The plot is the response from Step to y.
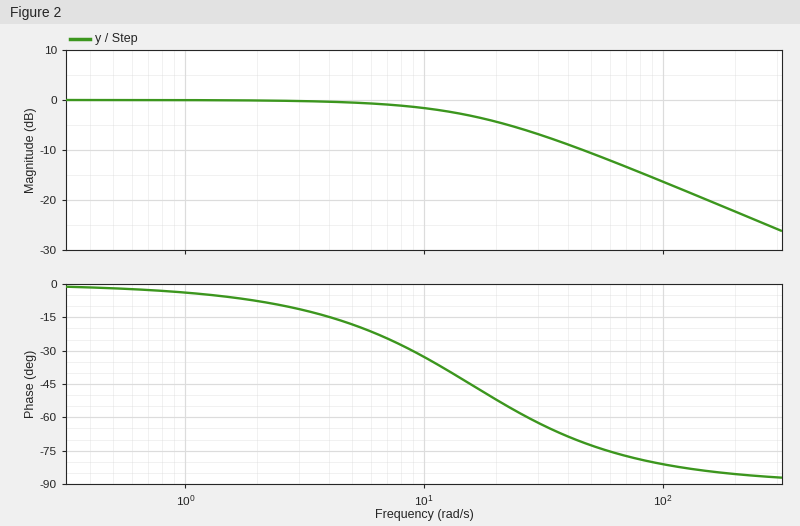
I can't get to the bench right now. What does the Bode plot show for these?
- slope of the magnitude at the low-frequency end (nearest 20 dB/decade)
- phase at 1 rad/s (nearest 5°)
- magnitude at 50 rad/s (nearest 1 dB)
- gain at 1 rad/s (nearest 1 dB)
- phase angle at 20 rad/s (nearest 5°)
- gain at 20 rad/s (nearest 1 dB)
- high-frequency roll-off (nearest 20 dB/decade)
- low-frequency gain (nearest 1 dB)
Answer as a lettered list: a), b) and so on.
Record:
a) 0 dB/decade
b) -5°
c) -11 dB
d) 0 dB
e) -50°
f) -4 dB
g) -20 dB/decade
h) 0 dB
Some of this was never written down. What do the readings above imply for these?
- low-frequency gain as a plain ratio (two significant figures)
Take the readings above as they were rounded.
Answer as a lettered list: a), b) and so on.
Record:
a) 1.0
